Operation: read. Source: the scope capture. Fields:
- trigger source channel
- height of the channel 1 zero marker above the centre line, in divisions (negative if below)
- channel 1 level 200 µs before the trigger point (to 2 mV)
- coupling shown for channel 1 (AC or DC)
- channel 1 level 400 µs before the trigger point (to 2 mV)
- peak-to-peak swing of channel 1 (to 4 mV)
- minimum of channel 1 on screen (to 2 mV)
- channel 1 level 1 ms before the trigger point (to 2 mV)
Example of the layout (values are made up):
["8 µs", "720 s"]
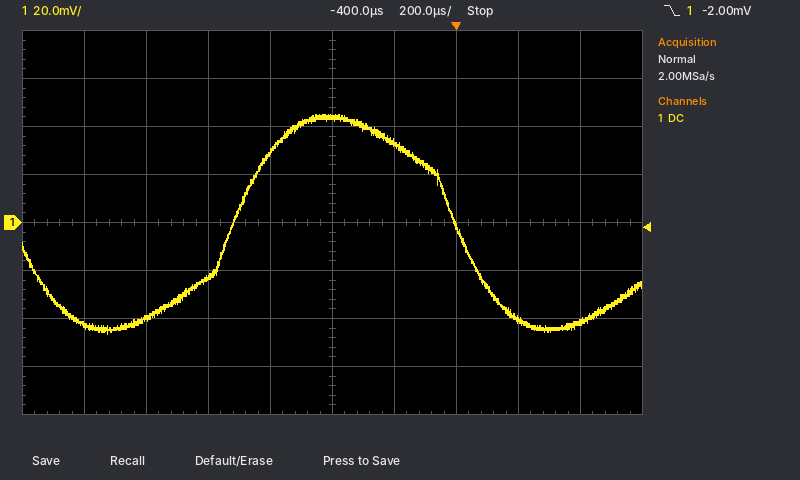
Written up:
["channel 1", "0.0 div", "32 mV", "DC", "44 mV", "92 mV", "-46 mV", "-40 mV"]
